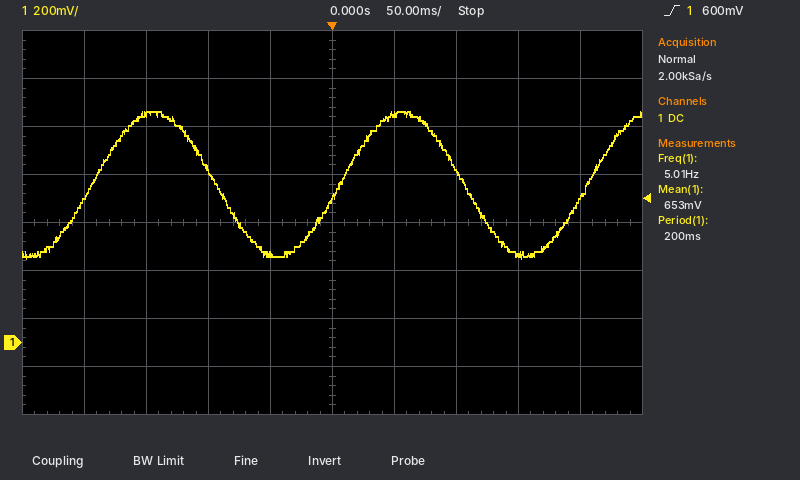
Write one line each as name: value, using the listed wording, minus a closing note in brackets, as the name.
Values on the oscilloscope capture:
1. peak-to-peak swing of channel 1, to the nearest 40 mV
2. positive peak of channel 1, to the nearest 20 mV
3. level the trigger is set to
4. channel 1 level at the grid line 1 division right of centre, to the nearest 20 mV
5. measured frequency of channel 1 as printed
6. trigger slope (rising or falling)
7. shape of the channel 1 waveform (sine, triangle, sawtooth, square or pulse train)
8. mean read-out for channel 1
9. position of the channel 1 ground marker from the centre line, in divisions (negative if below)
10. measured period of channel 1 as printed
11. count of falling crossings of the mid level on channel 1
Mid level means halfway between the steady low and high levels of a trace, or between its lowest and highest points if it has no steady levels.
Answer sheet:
peak-to-peak swing of channel 1, to the nearest 40 mV: 600 mV
positive peak of channel 1, to the nearest 20 mV: 960 mV
level the trigger is set to: 600 mV
channel 1 level at the grid line 1 division right of centre, to the nearest 20 mV: 960 mV
measured frequency of channel 1 as printed: 5.01 Hz
trigger slope: rising
shape of the channel 1 waveform: sine
mean read-out for channel 1: 653 mV
position of the channel 1 ground marker from the centre line, in divisions: -2.5 div
measured period of channel 1 as printed: 200 ms
count of falling crossings of the mid level on channel 1: 2
